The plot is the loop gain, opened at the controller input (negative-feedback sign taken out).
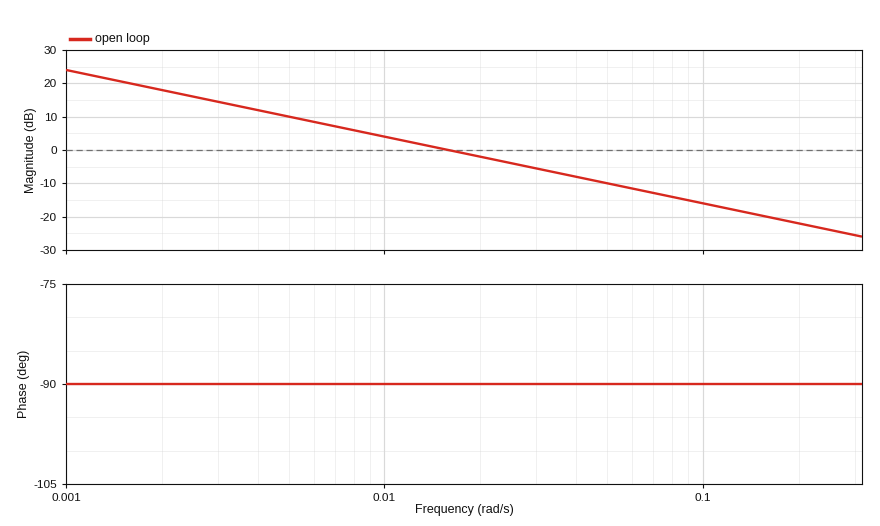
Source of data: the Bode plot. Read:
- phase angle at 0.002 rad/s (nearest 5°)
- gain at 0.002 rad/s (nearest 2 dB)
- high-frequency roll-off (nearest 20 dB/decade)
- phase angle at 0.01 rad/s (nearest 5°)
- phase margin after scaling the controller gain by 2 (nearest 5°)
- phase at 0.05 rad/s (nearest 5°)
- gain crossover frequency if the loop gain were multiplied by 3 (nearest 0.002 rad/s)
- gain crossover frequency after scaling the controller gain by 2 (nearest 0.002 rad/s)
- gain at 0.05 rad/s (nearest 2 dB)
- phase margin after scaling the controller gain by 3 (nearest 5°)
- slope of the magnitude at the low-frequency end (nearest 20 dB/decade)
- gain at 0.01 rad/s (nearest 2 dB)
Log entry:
-90°
18 dB
-20 dB/decade
-90°
90°
-90°
0.048 rad/s
0.032 rad/s
-10 dB
90°
-20 dB/decade
4 dB
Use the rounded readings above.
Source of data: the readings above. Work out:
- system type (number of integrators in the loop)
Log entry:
1
